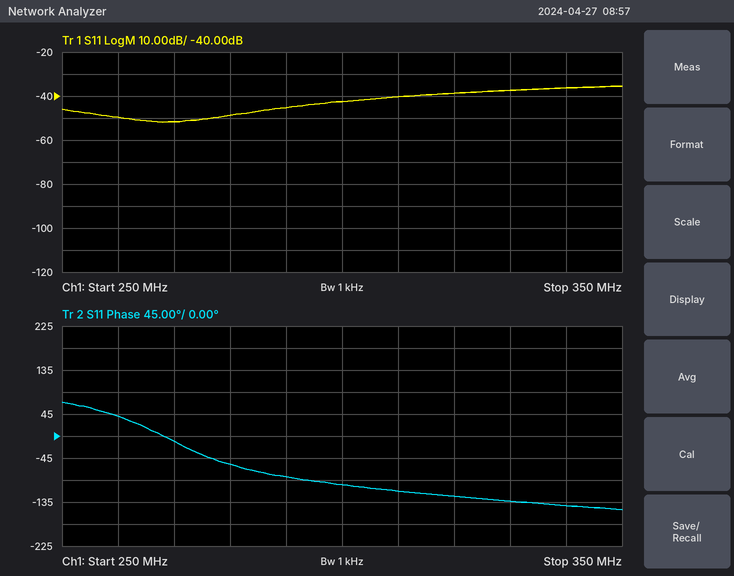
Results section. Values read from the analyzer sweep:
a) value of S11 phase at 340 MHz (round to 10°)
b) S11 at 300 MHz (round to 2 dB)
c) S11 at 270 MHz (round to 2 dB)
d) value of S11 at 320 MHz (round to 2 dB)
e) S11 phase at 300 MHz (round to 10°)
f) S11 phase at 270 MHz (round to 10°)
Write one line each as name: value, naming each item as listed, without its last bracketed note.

value of S11 phase at 340 MHz: -140°
S11 at 300 MHz: -42 dB
S11 at 270 MHz: -52 dB
value of S11 at 320 MHz: -38 dB
S11 phase at 300 MHz: -100°
S11 phase at 270 MHz: -10°
